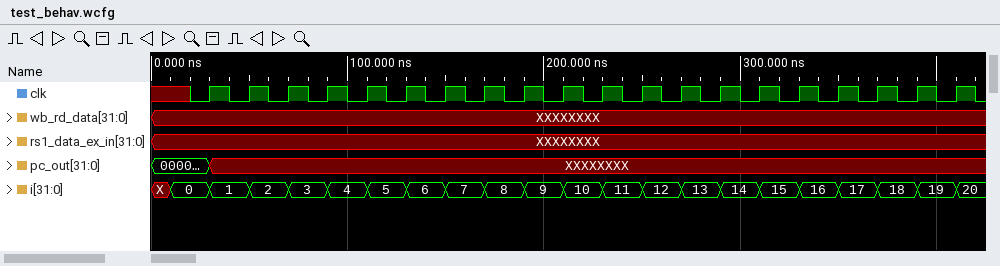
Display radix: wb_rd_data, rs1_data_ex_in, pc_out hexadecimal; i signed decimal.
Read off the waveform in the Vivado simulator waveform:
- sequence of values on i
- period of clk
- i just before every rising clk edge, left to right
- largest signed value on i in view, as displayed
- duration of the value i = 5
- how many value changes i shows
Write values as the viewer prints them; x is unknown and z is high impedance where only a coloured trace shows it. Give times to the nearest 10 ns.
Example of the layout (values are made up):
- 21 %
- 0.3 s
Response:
- X, 0, 1, 2, 3, 4, 5, 6, 7, 8, 9, 10, 11, 12, 13, 14, 15, 16, 17, 18, 19, 20
- 20 ns
- 0, 1, 2, 3, 4, 5, 6, 7, 8, 9, 10, 11, 12, 13, 14, 15, 16, 17, 18, 19
- 20
- 20 ns
- 21
